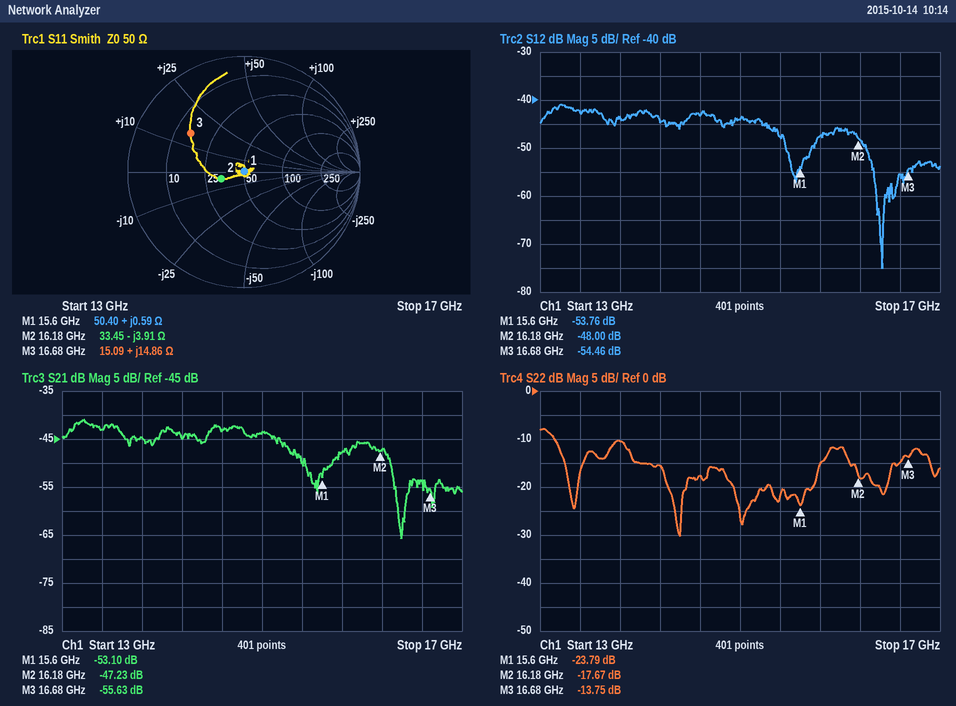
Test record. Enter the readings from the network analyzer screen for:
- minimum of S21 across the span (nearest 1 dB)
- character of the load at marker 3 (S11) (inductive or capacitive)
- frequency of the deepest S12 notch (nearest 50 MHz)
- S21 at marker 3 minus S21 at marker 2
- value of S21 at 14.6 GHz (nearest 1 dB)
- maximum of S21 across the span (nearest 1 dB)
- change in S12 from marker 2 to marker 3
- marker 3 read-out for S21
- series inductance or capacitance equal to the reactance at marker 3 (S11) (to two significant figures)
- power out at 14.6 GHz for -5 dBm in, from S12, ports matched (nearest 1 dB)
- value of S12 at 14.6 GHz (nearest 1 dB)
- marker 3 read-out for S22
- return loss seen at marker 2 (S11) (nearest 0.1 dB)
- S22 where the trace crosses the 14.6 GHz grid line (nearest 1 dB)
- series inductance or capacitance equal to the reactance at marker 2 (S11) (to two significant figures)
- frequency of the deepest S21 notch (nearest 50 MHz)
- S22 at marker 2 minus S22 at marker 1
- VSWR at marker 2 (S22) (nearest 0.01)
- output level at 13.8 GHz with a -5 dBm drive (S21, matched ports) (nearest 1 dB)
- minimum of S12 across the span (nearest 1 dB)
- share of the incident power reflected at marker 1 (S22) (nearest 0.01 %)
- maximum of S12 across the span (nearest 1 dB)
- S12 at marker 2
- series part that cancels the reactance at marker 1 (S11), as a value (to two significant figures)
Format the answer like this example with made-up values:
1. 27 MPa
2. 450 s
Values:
1. -66 dB
2. inductive
3. 16.40 GHz
4. -8.40 dB
5. -43 dB
6. -41 dB
7. -6.46 dB
8. -55.63 dB
9. 140 pH
10. -48 dBm
11. -43 dB
12. -13.75 dB
13. 13.8 dB
14. -18 dB
15. 2.5 pF
16. 16.40 GHz
17. 6.12 dB
18. 1.30
19. -50 dBm
20. -75 dB
21. 0.42 %
22. -41 dB
23. -48.00 dB
24. 17 pF
